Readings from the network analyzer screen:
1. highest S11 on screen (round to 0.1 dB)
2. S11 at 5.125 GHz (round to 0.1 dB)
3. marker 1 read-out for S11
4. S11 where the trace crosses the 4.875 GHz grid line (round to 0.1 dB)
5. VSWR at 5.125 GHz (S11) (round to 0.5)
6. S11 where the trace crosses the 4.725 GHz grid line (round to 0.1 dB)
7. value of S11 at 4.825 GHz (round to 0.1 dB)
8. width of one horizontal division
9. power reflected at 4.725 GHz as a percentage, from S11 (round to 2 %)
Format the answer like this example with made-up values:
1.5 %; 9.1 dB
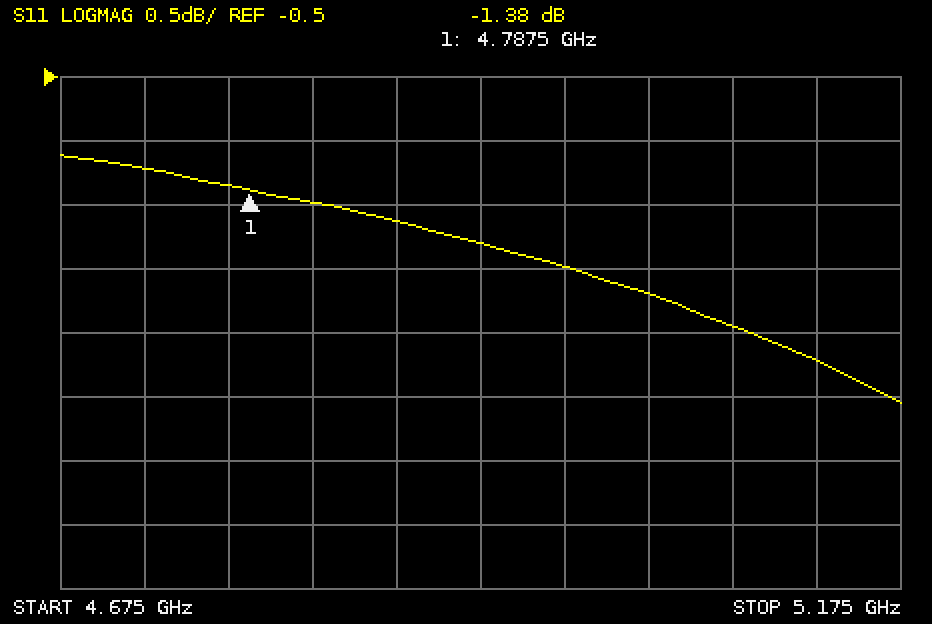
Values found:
-1.1 dB; -2.7 dB; -1.38 dB; -1.6 dB; 6.5; -1.2 dB; -1.5 dB; 50 MHz; 76 %
